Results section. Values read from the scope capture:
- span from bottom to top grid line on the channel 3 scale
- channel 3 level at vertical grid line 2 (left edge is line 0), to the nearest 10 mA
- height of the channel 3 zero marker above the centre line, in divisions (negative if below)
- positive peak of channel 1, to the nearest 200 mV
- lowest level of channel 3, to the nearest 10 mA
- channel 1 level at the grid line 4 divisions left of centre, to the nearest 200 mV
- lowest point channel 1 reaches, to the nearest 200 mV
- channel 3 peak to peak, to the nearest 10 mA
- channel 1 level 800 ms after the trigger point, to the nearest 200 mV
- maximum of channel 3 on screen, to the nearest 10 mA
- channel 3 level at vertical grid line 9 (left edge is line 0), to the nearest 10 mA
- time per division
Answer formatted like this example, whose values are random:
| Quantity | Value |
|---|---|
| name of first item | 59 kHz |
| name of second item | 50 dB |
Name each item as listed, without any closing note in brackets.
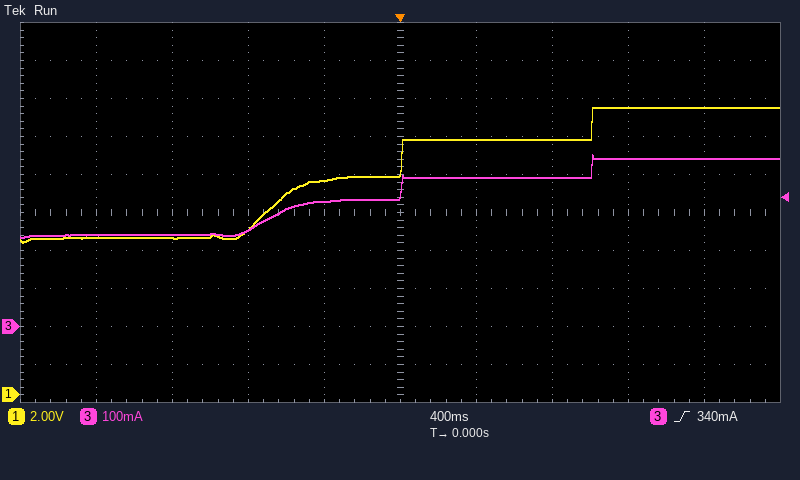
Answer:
| Quantity | Value |
|---|---|
| span from bottom to top grid line on the channel 3 scale | 1 A |
| channel 3 level at vertical grid line 2 (left edge is line 0), to the nearest 10 mA | 240 mA |
| height of the channel 3 zero marker above the centre line, in divisions | -3.0 div |
| positive peak of channel 1, to the nearest 200 mV | 15.2 V |
| lowest level of channel 3, to the nearest 10 mA | 230 mA |
| channel 1 level at the grid line 4 divisions left of centre, to the nearest 200 mV | 8.2 V |
| lowest point channel 1 reaches, to the nearest 200 mV | 8.0 V |
| channel 3 peak to peak, to the nearest 10 mA | 220 mA |
| channel 1 level 800 ms after the trigger point, to the nearest 200 mV | 13.4 V |
| maximum of channel 3 on screen, to the nearest 10 mA | 450 mA |
| channel 3 level at vertical grid line 9 (left edge is line 0), to the nearest 10 mA | 440 mA |
| time per division | 400 ms |
